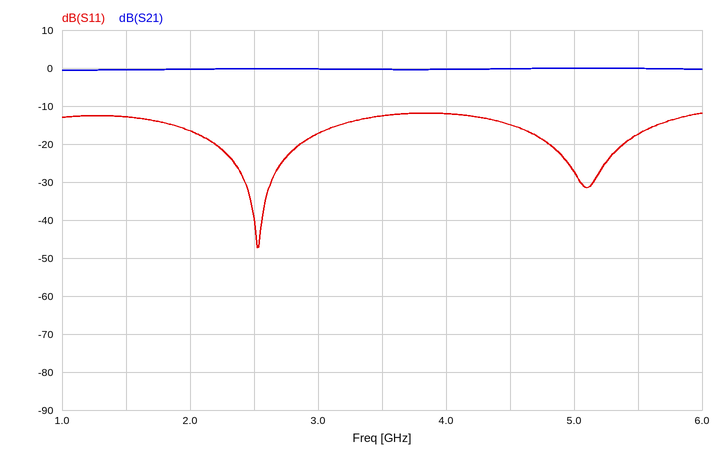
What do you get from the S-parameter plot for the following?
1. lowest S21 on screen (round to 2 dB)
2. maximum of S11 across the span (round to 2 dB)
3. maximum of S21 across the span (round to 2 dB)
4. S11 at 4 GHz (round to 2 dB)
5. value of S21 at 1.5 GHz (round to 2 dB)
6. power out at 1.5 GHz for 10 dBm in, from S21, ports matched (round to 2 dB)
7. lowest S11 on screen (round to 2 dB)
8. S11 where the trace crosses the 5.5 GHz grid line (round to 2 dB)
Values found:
0 dB
-12 dB
0 dB
-12 dB
0 dB
10 dBm
-48 dB
-18 dB
